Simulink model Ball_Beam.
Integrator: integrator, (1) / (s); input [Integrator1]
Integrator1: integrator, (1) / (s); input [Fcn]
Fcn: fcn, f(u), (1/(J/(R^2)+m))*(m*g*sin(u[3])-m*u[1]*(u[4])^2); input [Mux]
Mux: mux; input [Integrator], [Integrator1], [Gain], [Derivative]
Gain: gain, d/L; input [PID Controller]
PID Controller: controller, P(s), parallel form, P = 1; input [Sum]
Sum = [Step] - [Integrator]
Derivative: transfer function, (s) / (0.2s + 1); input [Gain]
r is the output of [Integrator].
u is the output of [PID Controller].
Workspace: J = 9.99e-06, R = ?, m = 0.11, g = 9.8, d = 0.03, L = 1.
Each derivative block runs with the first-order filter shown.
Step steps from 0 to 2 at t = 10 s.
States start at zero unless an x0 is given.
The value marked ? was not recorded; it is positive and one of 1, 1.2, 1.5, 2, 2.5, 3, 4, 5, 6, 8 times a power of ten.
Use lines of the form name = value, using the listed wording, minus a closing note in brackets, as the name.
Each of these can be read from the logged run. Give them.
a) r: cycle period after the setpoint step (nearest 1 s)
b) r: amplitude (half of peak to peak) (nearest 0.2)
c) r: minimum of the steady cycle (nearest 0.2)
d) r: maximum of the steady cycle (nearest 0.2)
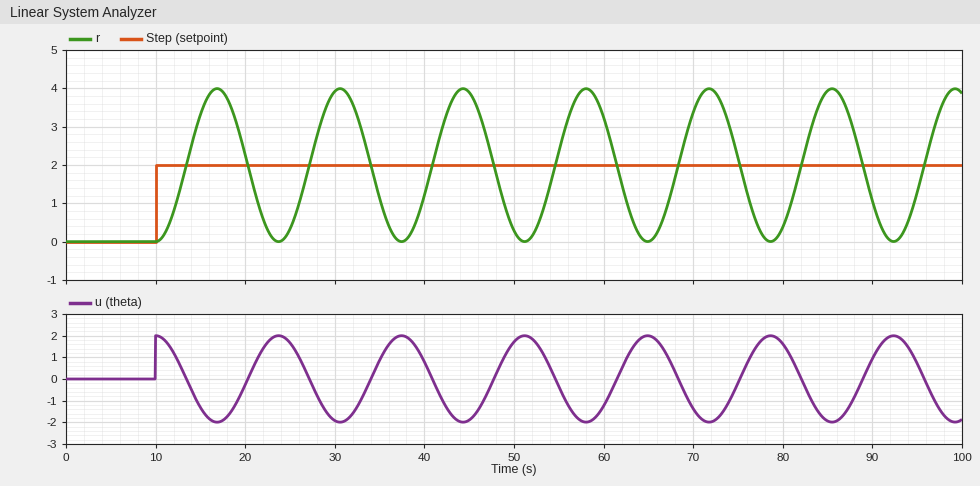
r: cycle period after the setpoint step = 14 s
r: amplitude (half of peak to peak) = 2.0
r: minimum of the steady cycle = 0.0
r: maximum of the steady cycle = 4.0
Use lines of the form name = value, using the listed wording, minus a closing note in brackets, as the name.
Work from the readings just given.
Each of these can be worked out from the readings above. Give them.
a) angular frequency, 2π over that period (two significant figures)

angular frequency, 2π over that period = 0.45 rad/s
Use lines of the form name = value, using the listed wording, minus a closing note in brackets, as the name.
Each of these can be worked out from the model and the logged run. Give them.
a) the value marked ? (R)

the value marked ? = 0.015
